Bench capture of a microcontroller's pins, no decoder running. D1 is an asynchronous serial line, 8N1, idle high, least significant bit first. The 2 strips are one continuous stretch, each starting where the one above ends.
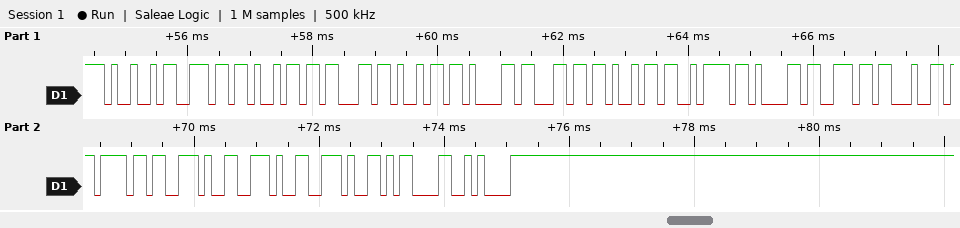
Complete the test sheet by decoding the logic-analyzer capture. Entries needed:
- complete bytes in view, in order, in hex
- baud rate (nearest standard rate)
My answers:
0x49 0x6E 0x69 0x63 0x69 0x61 0x6C 0x69 0x7A 0x61 0x6E 0x64 0x6F 0x2E 0x2E 0x2E 0x0D 0x0A
9600 baud
